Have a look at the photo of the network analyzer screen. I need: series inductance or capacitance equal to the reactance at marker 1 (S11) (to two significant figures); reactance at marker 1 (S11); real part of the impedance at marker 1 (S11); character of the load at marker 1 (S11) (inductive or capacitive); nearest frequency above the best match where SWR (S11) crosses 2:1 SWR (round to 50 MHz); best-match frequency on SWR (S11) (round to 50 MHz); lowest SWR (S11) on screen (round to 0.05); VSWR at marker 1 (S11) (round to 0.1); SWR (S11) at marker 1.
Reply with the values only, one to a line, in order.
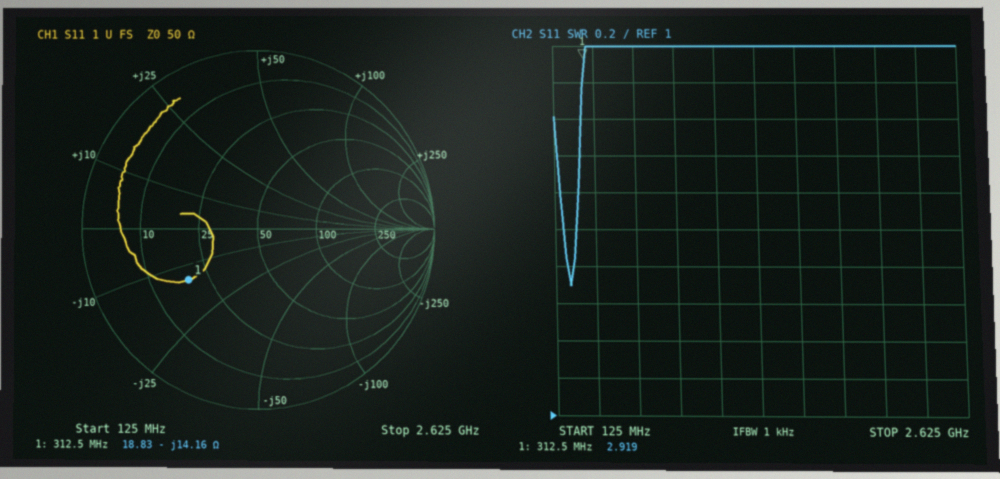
36 pF
-14.16 Ω
18.83 Ω
capacitive
250 MHz
200 MHz
1.70
2.9
2.919
